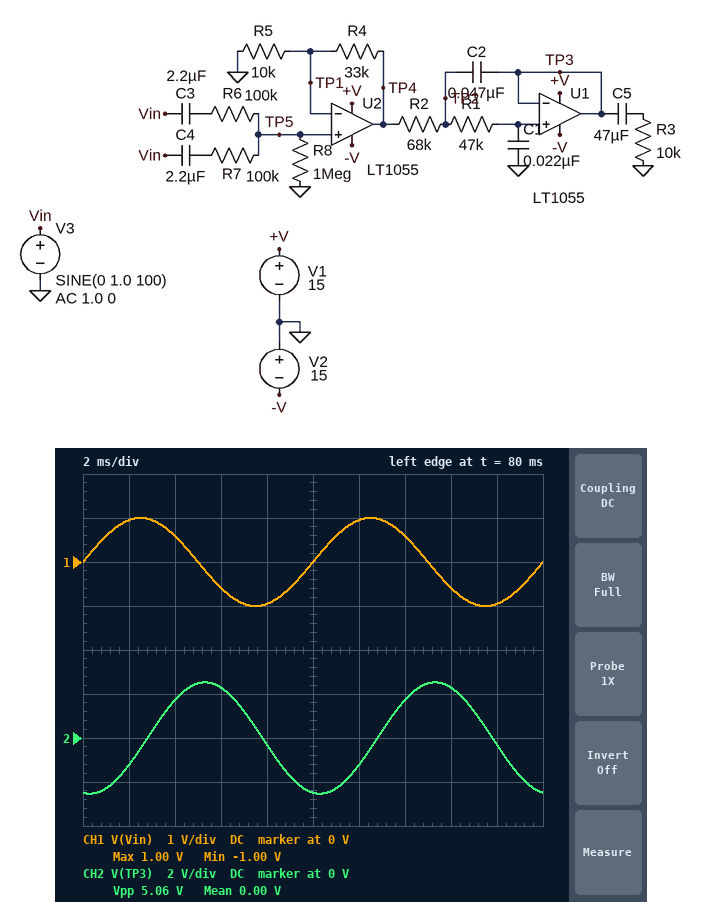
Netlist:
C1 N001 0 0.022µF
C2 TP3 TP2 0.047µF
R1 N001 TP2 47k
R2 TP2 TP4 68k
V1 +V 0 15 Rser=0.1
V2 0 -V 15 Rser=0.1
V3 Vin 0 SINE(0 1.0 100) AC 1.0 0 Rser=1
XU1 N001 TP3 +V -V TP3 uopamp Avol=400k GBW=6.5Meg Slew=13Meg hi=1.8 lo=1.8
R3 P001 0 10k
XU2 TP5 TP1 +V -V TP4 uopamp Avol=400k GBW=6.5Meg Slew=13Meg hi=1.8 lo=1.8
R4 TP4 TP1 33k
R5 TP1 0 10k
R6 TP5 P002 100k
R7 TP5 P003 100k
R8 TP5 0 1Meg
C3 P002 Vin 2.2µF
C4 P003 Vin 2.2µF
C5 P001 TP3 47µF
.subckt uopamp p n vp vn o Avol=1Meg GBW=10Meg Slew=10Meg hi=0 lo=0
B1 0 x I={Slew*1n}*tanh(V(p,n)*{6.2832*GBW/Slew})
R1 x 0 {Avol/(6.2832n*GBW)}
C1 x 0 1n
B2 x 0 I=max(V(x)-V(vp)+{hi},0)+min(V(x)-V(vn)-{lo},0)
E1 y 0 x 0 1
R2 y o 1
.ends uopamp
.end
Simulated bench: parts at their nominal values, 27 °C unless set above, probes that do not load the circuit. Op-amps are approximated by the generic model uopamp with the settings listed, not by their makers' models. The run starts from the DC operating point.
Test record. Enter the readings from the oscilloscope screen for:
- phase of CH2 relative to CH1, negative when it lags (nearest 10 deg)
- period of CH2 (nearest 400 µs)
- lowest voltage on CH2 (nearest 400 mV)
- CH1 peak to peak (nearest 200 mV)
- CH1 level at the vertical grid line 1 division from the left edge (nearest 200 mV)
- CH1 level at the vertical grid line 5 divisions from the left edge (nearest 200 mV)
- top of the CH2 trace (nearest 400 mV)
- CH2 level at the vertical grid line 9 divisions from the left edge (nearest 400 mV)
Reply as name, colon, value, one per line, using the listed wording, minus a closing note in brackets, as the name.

phase of CH2 relative to CH1, negative when it lags: -100 deg
period of CH2: 10.0 ms
lowest voltage on CH2: -2.4 V
CH1 peak to peak: 2.0 V
CH1 level at the vertical grid line 1 division from the left edge: 1.0 V
CH1 level at the vertical grid line 5 divisions from the left edge: 0 V
top of the CH2 trace: 2.4 V
CH2 level at the vertical grid line 9 divisions from the left edge: -400 mV
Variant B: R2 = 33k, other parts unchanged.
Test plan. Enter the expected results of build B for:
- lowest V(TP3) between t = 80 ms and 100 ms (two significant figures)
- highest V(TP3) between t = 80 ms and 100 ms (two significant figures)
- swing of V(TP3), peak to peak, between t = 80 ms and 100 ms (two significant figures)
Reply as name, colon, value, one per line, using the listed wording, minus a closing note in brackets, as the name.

lowest V(TP3) between t = 80 ms and 100 ms: -3.5 V
highest V(TP3) between t = 80 ms and 100 ms: 3.5 V
swing of V(TP3), peak to peak, between t = 80 ms and 100 ms: 7.0 V
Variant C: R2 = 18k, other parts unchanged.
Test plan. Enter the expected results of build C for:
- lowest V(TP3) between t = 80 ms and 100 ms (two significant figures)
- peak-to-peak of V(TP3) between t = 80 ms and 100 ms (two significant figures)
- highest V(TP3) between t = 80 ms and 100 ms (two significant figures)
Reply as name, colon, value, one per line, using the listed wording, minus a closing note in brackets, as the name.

lowest V(TP3) between t = 80 ms and 100 ms: -3.7 V
peak-to-peak of V(TP3) between t = 80 ms and 100 ms: 7.4 V
highest V(TP3) between t = 80 ms and 100 ms: 3.7 V
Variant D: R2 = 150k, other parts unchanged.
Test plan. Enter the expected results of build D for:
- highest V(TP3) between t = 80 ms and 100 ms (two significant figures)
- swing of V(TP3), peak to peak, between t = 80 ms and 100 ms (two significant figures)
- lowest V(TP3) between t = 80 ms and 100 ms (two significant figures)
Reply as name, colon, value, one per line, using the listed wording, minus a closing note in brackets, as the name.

highest V(TP3) between t = 80 ms and 100 ms: 1.2 V
swing of V(TP3), peak to peak, between t = 80 ms and 100 ms: 2.5 V
lowest V(TP3) between t = 80 ms and 100 ms: -1.2 V
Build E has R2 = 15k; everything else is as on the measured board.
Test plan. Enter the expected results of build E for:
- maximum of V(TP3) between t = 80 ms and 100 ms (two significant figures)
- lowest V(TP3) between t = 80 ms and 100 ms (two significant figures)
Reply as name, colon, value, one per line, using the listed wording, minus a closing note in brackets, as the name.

maximum of V(TP3) between t = 80 ms and 100 ms: 3.7 V
lowest V(TP3) between t = 80 ms and 100 ms: -3.7 V
